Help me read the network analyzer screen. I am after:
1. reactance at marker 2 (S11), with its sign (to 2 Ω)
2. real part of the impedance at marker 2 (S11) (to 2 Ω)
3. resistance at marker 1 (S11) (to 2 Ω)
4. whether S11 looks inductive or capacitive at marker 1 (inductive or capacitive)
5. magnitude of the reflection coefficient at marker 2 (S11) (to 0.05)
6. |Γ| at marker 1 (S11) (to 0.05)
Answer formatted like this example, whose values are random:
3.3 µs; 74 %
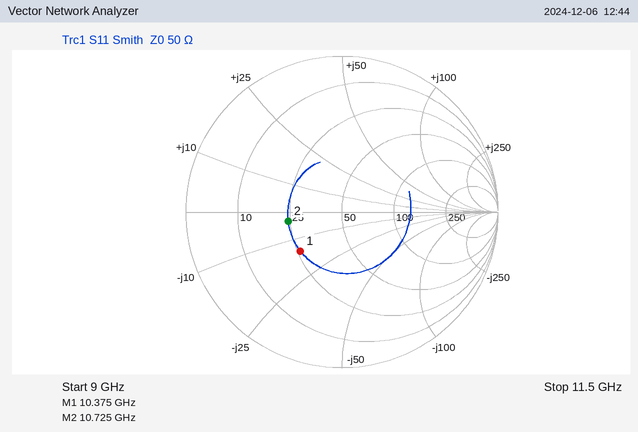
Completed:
-4 Ω; 24 Ω; 26 Ω; capacitive; 0.35; 0.35
